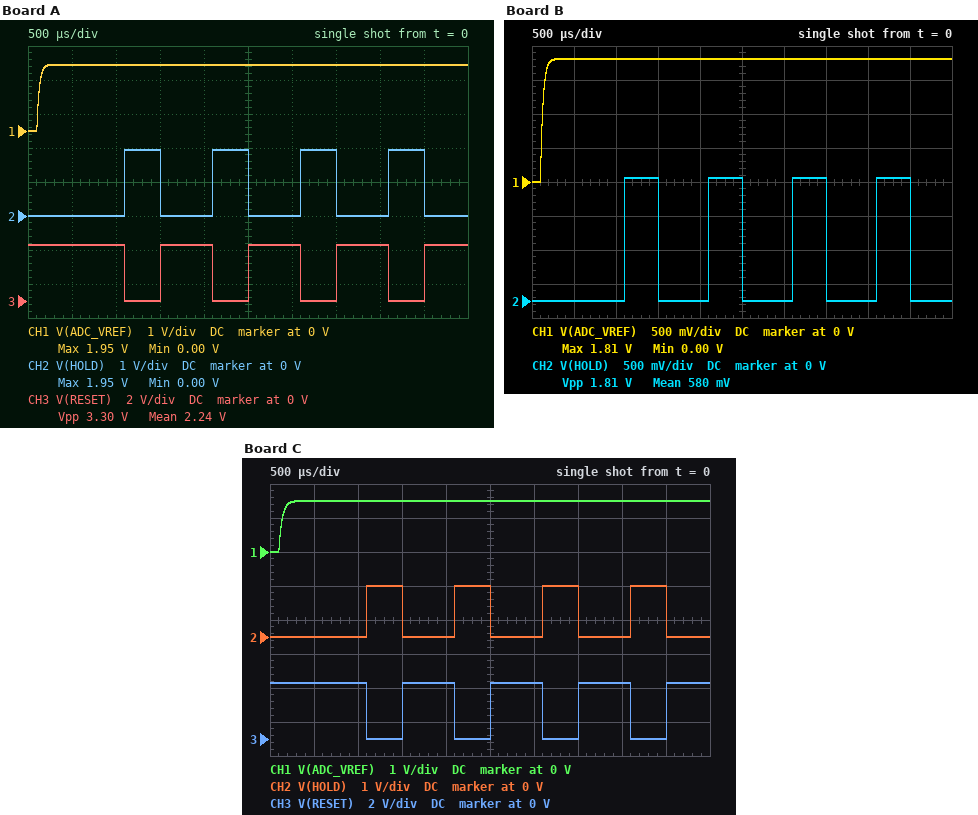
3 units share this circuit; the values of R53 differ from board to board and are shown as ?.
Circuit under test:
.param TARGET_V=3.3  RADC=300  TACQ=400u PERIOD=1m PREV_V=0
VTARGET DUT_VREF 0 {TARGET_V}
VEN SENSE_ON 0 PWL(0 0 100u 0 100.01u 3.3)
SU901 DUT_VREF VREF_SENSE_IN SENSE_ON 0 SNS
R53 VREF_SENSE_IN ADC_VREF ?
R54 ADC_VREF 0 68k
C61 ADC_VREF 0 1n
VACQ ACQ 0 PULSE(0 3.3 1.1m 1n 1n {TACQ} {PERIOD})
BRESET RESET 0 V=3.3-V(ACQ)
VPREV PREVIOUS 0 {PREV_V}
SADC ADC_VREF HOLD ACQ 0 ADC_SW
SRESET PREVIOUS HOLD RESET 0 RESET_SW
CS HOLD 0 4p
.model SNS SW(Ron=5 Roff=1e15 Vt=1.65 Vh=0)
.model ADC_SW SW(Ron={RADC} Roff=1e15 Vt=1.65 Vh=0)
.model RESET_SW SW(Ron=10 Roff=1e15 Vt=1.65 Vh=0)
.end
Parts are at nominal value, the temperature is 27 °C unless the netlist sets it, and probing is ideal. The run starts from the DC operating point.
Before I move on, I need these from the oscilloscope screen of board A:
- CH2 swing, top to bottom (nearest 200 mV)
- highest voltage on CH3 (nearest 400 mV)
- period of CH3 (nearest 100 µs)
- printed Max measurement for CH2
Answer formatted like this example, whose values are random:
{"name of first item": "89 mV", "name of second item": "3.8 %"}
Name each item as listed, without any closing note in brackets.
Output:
{"CH2 swing, top to bottom": "2.0 V", "highest voltage on CH3": "3.2 V", "period of CH3": "1.0 ms", "printed Max measurement for CH2": "1.95 V"}
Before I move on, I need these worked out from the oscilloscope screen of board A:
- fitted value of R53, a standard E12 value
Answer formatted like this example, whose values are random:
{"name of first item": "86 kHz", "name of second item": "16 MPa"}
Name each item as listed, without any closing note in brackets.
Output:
{"fitted value of R53, a standard E12 value": "47 kΩ"}
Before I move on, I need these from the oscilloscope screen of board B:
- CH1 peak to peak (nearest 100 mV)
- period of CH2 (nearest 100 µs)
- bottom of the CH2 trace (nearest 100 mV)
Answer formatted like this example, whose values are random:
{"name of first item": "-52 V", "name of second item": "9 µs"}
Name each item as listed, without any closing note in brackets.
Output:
{"CH1 peak to peak": "1.8 V", "period of CH2": "1.0 ms", "bottom of the CH2 trace": "0 V"}
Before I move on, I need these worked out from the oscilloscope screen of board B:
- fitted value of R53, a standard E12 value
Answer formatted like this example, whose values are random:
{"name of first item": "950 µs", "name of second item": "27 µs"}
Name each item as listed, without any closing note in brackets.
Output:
{"fitted value of R53, a standard E12 value": "56 kΩ"}
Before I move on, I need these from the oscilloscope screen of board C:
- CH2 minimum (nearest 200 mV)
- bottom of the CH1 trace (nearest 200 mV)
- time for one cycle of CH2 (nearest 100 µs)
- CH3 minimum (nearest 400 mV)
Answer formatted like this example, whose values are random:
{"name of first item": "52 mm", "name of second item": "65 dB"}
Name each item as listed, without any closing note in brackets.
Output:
{"CH2 minimum": "0 V", "bottom of the CH1 trace": "0 V", "time for one cycle of CH2": "1.0 ms", "CH3 minimum": "0 V"}
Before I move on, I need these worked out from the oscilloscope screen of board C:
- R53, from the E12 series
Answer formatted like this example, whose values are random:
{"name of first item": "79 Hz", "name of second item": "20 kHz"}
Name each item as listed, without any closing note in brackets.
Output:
{"R53, from the E12 series": "82 kΩ"}
